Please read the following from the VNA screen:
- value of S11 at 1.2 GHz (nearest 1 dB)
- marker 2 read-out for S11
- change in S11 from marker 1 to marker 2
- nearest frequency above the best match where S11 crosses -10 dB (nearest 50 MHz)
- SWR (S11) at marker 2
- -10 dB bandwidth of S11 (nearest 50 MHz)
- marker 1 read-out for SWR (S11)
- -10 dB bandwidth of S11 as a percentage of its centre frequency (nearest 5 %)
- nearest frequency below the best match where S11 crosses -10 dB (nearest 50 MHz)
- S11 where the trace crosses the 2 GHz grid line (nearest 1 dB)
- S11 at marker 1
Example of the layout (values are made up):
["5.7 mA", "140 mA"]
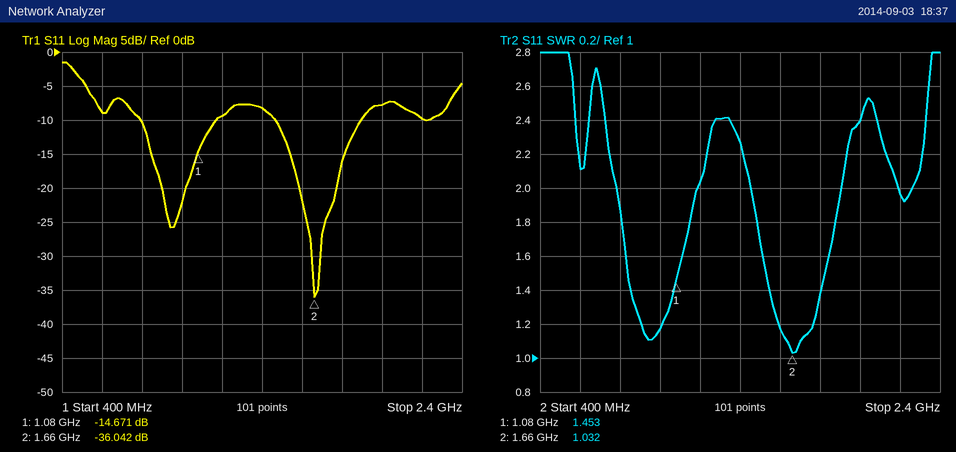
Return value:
["-9 dB", "-36.042 dB", "-21.371 dB", "1.90 GHz", "1.032", "450 MHz", "1.453", "25 %", "1.45 GHz", "-8 dB", "-14.671 dB"]
